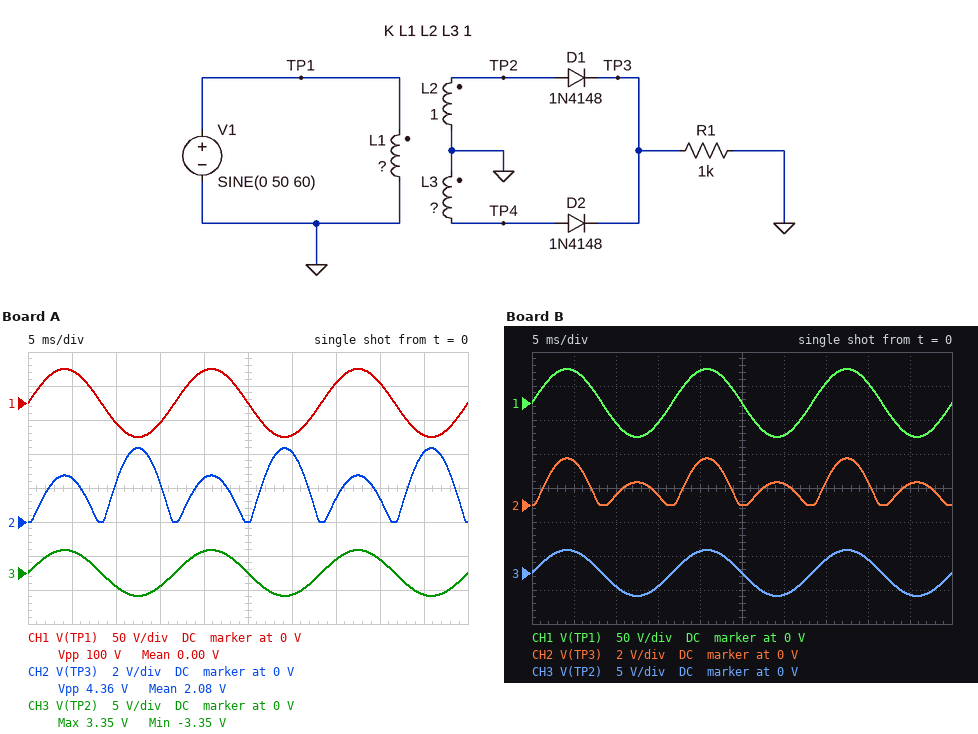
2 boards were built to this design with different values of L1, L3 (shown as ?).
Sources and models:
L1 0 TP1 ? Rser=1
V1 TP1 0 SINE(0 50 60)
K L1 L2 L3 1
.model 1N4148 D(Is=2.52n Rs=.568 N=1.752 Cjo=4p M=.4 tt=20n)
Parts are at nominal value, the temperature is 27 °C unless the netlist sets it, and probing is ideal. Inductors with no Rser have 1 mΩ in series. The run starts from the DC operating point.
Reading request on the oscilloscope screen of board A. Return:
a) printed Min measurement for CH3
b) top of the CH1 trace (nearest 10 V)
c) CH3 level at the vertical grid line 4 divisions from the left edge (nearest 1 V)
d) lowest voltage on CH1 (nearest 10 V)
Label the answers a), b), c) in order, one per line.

a) -3.35 V
b) 50 V
c) 3 V
d) -50 V
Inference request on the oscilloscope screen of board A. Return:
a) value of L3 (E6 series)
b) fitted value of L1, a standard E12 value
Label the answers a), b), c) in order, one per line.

a) 2.2 H
b) 220 H
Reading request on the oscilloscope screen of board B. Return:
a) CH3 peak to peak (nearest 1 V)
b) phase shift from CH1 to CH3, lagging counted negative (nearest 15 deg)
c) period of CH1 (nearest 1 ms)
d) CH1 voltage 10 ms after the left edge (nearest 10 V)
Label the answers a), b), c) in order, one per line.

a) 7 V
b) 0 deg
c) 17 ms
d) -30 V
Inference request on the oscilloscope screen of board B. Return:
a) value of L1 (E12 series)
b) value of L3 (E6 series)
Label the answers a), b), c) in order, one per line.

a) 220 H
b) 330 mH
